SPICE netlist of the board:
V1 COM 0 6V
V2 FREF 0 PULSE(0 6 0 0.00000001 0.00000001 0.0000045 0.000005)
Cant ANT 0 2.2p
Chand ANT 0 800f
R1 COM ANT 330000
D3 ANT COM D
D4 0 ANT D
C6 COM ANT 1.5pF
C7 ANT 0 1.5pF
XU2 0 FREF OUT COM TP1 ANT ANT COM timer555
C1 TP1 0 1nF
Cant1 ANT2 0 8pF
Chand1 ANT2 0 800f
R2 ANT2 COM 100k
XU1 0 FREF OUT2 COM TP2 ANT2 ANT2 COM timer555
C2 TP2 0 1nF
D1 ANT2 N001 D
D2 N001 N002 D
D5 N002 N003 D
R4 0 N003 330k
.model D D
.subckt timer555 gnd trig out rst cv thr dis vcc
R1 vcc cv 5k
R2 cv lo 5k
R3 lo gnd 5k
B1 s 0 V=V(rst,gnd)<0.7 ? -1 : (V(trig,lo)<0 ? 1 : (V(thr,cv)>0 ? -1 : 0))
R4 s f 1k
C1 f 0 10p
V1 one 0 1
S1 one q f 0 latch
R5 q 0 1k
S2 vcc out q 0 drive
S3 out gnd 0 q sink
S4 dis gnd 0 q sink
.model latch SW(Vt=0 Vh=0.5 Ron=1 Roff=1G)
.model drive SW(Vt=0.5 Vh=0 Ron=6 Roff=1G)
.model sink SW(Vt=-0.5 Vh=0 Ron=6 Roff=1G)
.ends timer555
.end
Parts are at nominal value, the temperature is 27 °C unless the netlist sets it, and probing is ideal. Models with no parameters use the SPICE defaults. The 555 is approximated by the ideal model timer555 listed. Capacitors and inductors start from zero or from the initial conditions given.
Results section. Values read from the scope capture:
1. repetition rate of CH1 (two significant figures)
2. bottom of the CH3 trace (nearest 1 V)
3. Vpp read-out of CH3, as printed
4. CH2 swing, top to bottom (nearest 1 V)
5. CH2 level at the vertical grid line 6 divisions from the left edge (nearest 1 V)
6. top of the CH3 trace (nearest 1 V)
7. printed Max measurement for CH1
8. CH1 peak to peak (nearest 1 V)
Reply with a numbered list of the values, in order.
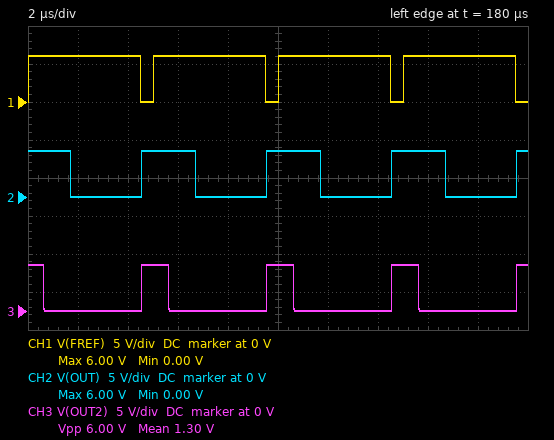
1. 200 kHz
2. 0 V
3. 6.00 V
4. 6 V
5. 0 V
6. 6 V
7. 6.00 V
8. 6 V
